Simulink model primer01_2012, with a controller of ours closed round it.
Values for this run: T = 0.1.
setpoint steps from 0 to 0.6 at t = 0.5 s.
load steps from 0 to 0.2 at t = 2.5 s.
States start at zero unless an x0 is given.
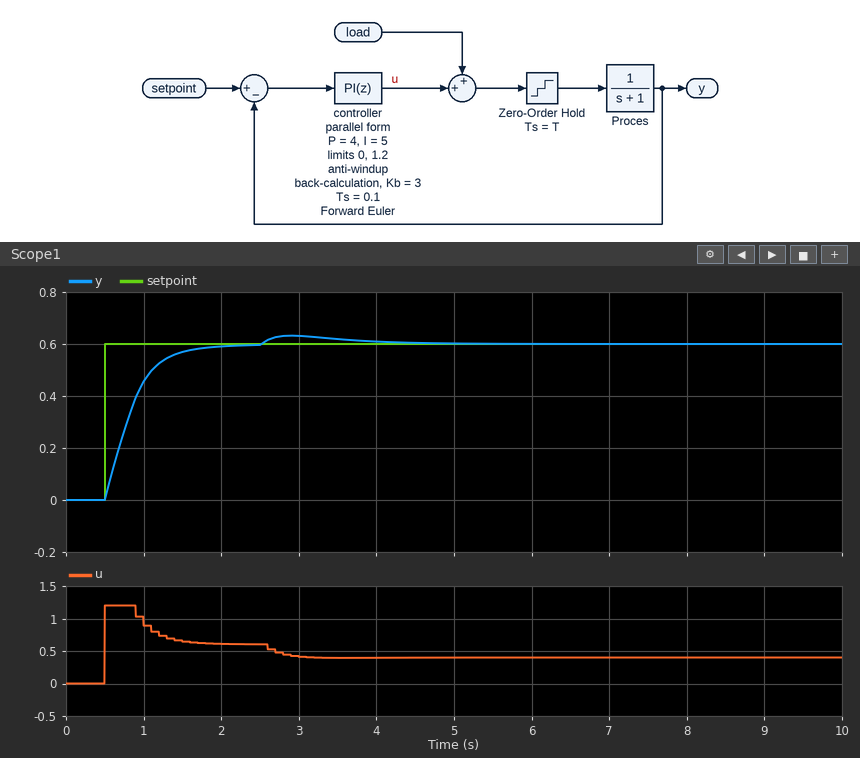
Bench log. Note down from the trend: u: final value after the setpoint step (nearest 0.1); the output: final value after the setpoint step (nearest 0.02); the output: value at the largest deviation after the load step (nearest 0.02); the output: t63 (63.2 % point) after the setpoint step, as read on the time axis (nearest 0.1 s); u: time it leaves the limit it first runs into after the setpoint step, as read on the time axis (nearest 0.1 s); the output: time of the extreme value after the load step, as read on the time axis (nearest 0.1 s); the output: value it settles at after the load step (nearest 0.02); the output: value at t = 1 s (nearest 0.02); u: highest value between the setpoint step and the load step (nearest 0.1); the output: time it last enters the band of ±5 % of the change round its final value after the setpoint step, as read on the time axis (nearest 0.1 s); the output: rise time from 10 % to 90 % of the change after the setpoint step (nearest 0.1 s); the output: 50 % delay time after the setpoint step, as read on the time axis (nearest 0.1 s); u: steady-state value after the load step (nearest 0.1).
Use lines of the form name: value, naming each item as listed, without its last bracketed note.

u: final value after the setpoint step: 0.6
the output: final value after the setpoint step: 0.60
the output: value at the largest deviation after the load step: 0.64
the output: t63 (63.2 % point) after the setpoint step, as read on the time axis: 0.9 s
u: time it leaves the limit it first runs into after the setpoint step, as read on the time axis: 0.9 s
the output: time of the extreme value after the load step, as read on the time axis: 2.9 s
the output: value it settles at after the load step: 0.60
the output: value at t = 1 s: 0.46
u: highest value between the setpoint step and the load step: 1.2
the output: time it last enters the band of ±5 % of the change round its final value after the setpoint step, as read on the time axis: 1.5 s
the output: rise time from 10 % to 90 % of the change after the setpoint step: 0.7 s
the output: 50 % delay time after the setpoint step, as read on the time axis: 0.8 s
u: steady-state value after the load step: 0.4
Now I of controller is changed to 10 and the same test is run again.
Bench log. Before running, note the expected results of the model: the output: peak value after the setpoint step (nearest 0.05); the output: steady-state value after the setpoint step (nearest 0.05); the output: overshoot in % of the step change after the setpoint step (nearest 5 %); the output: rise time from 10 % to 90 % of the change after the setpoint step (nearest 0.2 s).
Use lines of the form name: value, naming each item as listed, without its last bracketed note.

the output: peak value after the setpoint step: 0.65
the output: steady-state value after the setpoint step: 0.60
the output: overshoot in % of the step change after the setpoint step: 10 %
the output: rise time from 10 % to 90 % of the change after the setpoint step: 0.6 s
